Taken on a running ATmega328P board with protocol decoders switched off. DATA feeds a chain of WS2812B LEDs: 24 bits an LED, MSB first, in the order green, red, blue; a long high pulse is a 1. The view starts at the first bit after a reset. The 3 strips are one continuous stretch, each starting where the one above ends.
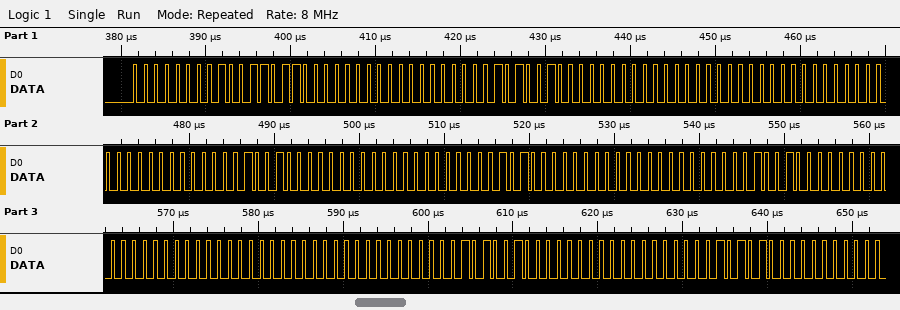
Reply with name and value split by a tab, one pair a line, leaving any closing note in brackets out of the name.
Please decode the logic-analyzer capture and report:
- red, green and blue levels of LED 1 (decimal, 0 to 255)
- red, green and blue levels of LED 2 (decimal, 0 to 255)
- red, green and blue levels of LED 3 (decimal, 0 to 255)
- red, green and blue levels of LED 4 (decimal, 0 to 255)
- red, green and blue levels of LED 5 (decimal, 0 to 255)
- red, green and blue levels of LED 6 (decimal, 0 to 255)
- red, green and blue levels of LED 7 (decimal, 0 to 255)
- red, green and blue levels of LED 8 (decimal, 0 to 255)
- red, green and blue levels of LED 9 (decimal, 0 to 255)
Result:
red, green and blue levels of LED 1	155, 0, 0
red, green and blue levels of LED 2	41, 0, 0
red, green and blue levels of LED 3	0, 0, 0
red, green and blue levels of LED 4	9, 0, 0
red, green and blue levels of LED 5	10, 0, 0
red, green and blue levels of LED 6	9, 0, 0
red, green and blue levels of LED 7	0, 0, 0
red, green and blue levels of LED 8	41, 0, 0
red, green and blue levels of LED 9	42, 0, 0
